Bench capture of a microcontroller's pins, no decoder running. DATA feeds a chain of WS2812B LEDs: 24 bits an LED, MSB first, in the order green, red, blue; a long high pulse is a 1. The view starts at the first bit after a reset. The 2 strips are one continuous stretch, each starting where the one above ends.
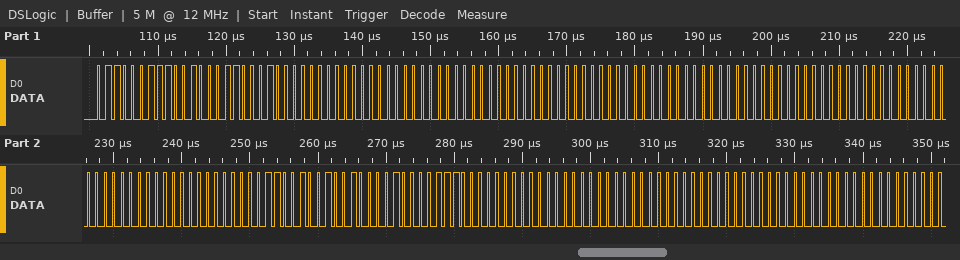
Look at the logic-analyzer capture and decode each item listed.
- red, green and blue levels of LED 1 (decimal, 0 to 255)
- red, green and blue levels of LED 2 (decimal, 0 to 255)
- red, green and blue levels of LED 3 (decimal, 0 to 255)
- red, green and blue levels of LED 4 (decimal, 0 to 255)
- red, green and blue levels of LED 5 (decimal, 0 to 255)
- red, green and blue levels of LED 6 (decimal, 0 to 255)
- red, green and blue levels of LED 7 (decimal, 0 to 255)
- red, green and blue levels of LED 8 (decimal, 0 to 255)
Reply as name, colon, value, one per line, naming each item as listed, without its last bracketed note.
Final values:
red, green and blue levels of LED 1: 145, 99, 136
red, green and blue levels of LED 2: 0, 0, 0
red, green and blue levels of LED 3: 0, 0, 0
red, green and blue levels of LED 4: 0, 0, 0
red, green and blue levels of LED 5: 0, 0, 0
red, green and blue levels of LED 6: 144, 100, 135
red, green and blue levels of LED 7: 0, 0, 0
red, green and blue levels of LED 8: 0, 0, 0
